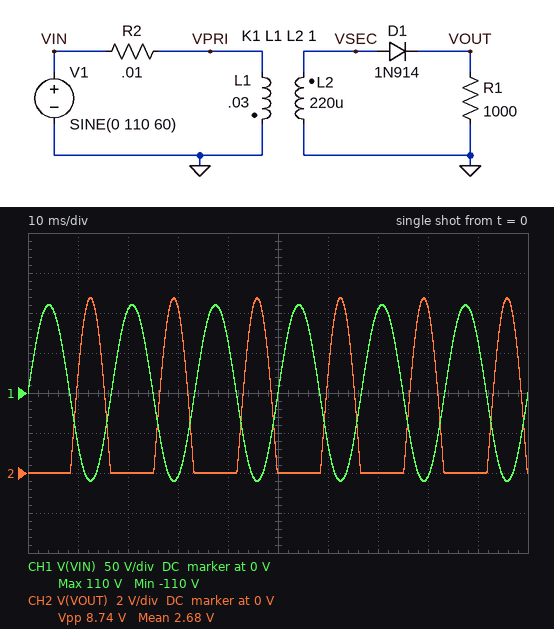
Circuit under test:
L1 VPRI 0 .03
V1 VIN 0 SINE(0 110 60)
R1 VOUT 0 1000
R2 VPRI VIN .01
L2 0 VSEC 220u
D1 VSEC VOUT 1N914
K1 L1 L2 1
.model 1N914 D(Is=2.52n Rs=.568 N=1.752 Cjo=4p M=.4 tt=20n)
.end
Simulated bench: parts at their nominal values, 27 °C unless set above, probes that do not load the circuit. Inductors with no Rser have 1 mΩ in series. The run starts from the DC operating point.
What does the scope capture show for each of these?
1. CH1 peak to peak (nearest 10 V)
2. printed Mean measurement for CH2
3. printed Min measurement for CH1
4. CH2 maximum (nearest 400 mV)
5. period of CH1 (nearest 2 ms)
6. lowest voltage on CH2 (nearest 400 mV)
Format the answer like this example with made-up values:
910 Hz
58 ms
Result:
220 V
2.68 V
-110 V
8.8 V
16 ms
0 V
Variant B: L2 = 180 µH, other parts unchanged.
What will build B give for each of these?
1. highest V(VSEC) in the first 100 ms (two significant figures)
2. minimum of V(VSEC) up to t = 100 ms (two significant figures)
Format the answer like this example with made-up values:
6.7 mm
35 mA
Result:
8.5 V
-8.5 V
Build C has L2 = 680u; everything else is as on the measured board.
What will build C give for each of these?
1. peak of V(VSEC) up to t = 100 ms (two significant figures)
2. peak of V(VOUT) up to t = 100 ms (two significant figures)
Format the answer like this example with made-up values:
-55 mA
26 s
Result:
17 V
16 V
